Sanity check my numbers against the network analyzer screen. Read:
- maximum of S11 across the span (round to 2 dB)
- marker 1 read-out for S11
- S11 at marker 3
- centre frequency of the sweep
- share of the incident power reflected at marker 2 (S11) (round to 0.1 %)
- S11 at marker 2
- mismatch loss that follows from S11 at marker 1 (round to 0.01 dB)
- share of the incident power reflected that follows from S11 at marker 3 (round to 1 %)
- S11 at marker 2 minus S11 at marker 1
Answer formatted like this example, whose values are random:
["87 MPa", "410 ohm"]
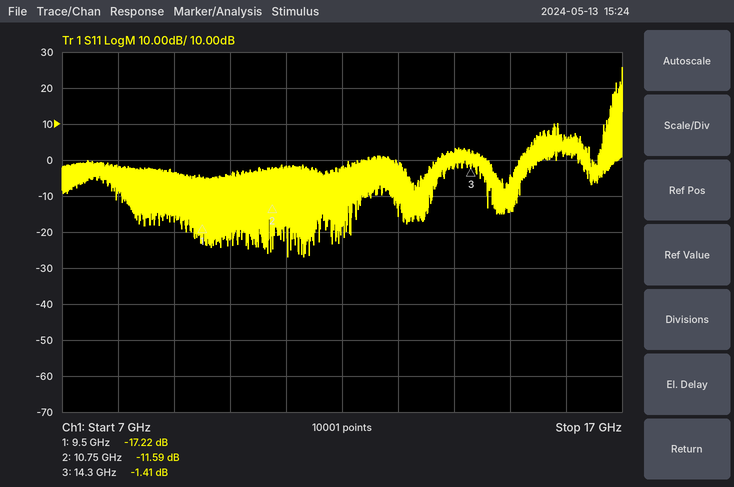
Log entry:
["26 dB", "-17.22 dB", "-1.41 dB", "12 GHz", "6.9 %", "-11.59 dB", "0.08 dB", "72 %", "5.63 dB"]
